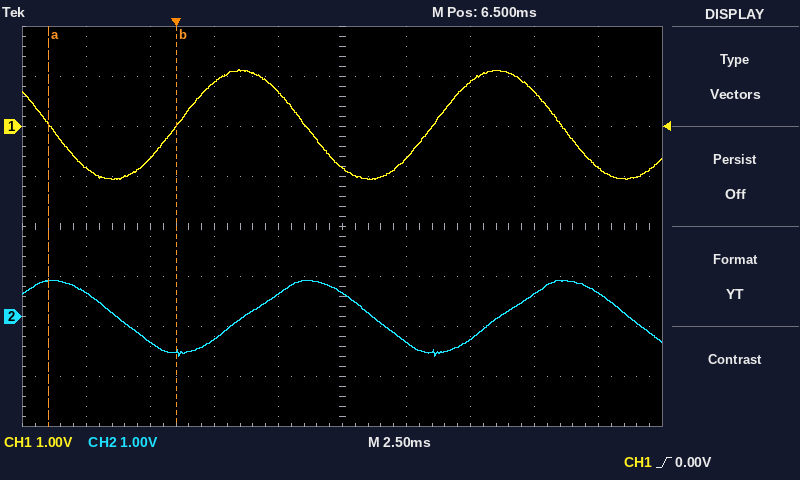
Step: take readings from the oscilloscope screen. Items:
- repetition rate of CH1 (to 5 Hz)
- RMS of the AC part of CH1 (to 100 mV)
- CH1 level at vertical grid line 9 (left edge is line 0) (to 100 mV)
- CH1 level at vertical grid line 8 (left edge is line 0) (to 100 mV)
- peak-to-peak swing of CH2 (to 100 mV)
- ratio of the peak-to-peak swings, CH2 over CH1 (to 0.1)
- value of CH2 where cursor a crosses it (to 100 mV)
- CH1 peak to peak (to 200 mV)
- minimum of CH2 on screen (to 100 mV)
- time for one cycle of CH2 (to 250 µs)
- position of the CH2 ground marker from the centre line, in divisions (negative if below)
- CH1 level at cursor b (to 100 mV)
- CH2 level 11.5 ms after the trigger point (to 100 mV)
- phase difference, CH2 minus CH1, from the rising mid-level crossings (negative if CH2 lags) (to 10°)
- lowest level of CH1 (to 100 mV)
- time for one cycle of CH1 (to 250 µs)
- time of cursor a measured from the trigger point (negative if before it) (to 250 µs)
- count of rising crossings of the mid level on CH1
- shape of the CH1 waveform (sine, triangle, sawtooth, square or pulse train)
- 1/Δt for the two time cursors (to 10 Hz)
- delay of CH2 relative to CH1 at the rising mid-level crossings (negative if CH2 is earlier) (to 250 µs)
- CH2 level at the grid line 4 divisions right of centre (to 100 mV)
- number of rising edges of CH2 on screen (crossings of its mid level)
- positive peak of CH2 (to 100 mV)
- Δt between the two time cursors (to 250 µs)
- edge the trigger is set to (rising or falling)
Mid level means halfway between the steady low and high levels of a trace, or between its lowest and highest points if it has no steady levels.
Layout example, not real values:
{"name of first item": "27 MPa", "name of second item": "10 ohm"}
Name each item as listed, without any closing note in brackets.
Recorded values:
{"repetition rate of CH1": "100 Hz", "RMS of the AC part of CH1": "800 mV", "CH1 level at vertical grid line 9 (left edge is line 0)": "-800 mV", "CH1 level at vertical grid line 8 (left edge is line 0)": "700 mV", "peak-to-peak swing of CH2": "1.5 V", "ratio of the peak-to-peak swings, CH2 over CH1": "0.7", "value of CH2 where cursor a crosses it": "700 mV", "CH1 peak to peak": "2.2 V", "minimum of CH2 on screen": "-800 mV", "time for one cycle of CH2": "10.00 ms", "position of the CH2 ground marker from the centre line, in divisions": "-1.8 div", "CH1 level at cursor b": "0.0 V", "CH2 level 11.5 ms after the trigger point": "-500 mV", "phase difference, CH2 minus CH1, from the rising mid-level crossings (negative if CH2 lags)": "-90°", "lowest level of CH1": "-1.1 V", "time for one cycle of CH1": "10.00 ms", "time of cursor a measured from the trigger point (negative if before it)": "-5.00 ms", "count of rising crossings of the mid level on CH1": "2", "shape of the CH1 waveform": "sine", "1/Δt for the two time cursors": "200 Hz", "delay of CH2 relative to CH1 at the rising mid-level crossings (negative if CH2 is earlier)": "+2.50 ms", "CH2 level at the grid line 4 divisions right of centre": "500 mV", "number of rising edges of CH2 on screen": "2", "positive peak of CH2": "700 mV", "Δt between the two time cursors": "5.00 ms", "edge the trigger is set to": "rising"}
